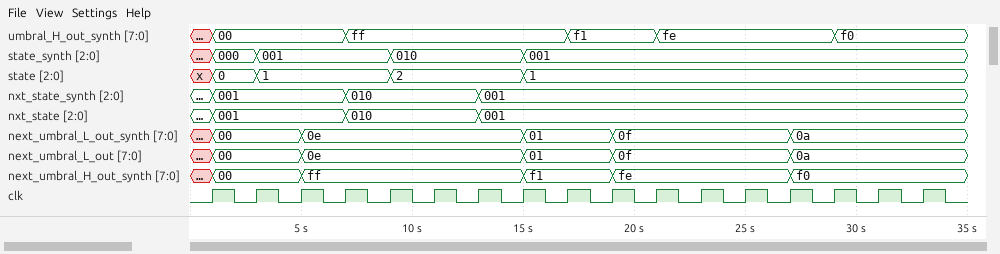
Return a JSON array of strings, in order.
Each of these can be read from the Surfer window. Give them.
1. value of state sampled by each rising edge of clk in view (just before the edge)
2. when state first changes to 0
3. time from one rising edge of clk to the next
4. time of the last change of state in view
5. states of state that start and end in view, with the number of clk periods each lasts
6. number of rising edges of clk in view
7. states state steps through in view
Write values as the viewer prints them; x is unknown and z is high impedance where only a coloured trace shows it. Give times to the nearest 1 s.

["x, 0, 1, 1, 1, 2, 2, 2, 1, 1, 1, 1, 1, 1, 1, 1, 1", "1 s", "2 s", "15 s", "0: 1, 1: 3, 2: 3", "17", "x, 0, 1, 2, 1"]
